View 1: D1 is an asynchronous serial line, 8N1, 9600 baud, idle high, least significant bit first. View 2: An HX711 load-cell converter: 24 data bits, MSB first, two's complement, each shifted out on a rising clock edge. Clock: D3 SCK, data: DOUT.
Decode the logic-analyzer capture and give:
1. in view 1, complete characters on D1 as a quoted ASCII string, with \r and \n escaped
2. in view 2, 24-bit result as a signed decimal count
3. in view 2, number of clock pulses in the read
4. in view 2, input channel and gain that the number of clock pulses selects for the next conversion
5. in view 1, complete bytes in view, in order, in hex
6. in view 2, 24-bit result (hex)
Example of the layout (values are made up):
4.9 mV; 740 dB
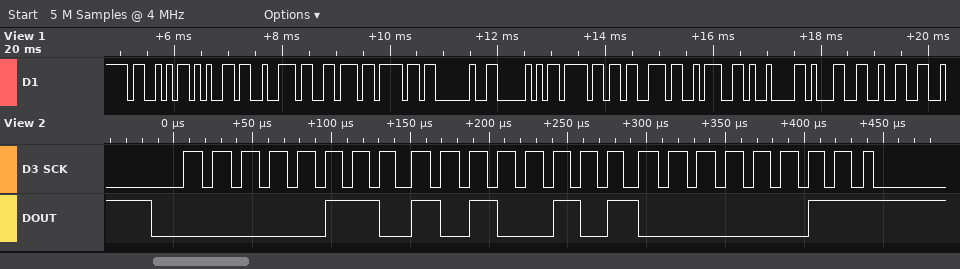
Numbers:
"Servo Pos:\t12"; 435459; 25; channel A, gain 128; 53 65 72 76 6F 20 50 6F 73 3A 09 31 32; 0x06A503
